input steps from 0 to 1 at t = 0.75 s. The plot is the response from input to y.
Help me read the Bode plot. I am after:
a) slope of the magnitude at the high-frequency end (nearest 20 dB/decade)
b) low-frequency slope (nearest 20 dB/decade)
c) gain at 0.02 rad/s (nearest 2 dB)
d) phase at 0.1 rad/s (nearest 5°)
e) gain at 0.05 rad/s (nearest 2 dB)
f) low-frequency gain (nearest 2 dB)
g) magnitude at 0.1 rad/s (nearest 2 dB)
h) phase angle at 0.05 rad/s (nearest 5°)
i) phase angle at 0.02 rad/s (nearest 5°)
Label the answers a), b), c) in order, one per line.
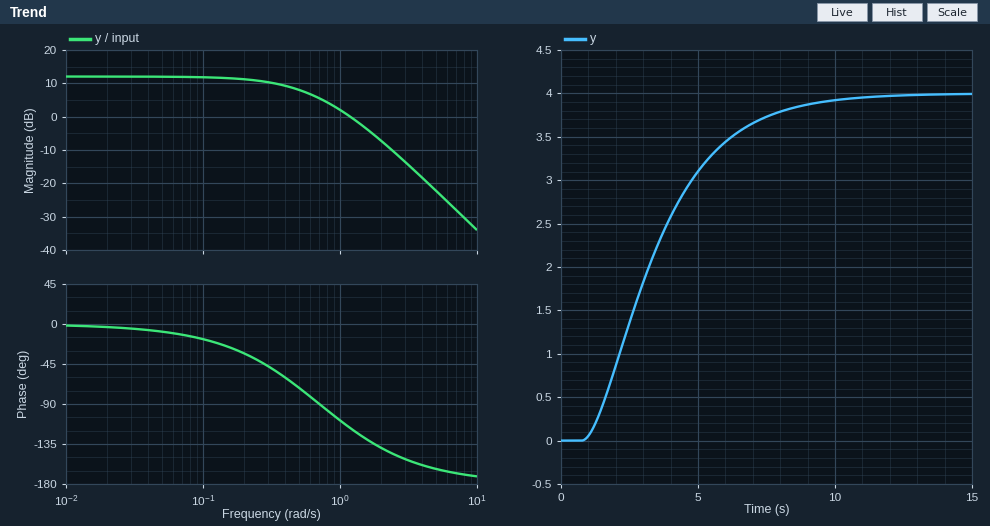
a) -40 dB/decade
b) 0 dB/decade
c) 12 dB
d) -15°
e) 12 dB
f) 12 dB
g) 12 dB
h) -10°
i) -5°
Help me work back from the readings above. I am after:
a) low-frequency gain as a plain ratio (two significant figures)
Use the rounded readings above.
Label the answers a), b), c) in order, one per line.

a) 4.0
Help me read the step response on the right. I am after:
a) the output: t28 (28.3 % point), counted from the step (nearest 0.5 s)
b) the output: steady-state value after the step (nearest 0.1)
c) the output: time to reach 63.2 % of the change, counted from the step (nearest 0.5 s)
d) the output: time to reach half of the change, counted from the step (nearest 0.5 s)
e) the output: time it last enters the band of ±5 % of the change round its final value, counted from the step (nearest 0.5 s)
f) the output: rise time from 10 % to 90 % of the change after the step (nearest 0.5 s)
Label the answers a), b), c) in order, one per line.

a) 1.5 s
b) 4.0
c) 3.0 s
d) 2.5 s
e) 7.5 s
f) 5.0 s
